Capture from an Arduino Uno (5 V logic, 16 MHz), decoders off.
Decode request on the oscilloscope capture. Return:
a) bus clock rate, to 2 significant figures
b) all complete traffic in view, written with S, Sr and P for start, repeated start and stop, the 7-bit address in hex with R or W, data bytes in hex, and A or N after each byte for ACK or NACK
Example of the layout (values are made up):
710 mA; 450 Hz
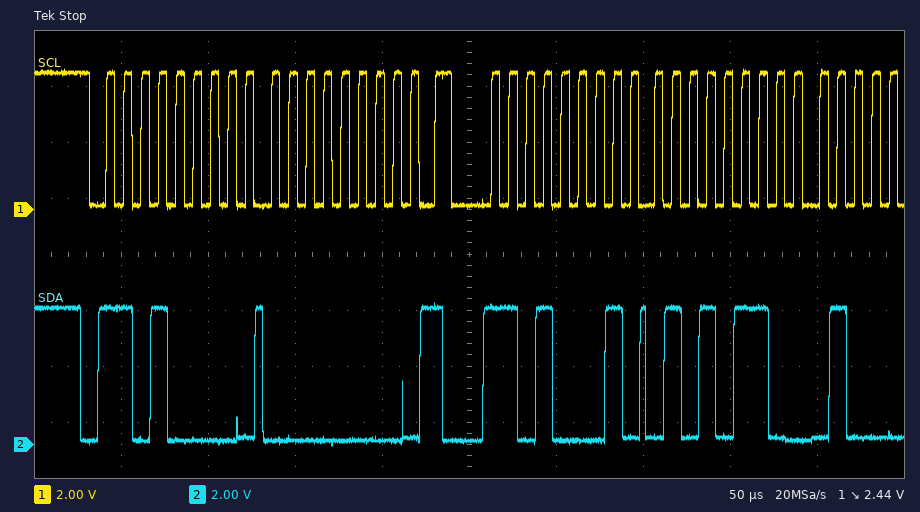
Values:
100 kHz; S 68W A 00 A Sr 68R A 56 A
